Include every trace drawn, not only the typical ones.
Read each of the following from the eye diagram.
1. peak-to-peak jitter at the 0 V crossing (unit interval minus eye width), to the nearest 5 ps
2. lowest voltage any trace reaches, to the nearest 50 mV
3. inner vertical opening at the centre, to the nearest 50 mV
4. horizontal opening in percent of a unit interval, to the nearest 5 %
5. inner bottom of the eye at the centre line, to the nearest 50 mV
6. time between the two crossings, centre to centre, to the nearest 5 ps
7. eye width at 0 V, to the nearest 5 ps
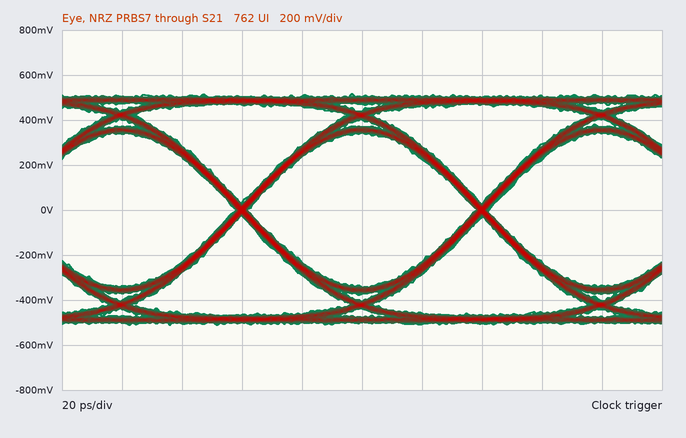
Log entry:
5 ps
-500 mV
700 mV
95 %
-350 mV
80 ps
75 ps
